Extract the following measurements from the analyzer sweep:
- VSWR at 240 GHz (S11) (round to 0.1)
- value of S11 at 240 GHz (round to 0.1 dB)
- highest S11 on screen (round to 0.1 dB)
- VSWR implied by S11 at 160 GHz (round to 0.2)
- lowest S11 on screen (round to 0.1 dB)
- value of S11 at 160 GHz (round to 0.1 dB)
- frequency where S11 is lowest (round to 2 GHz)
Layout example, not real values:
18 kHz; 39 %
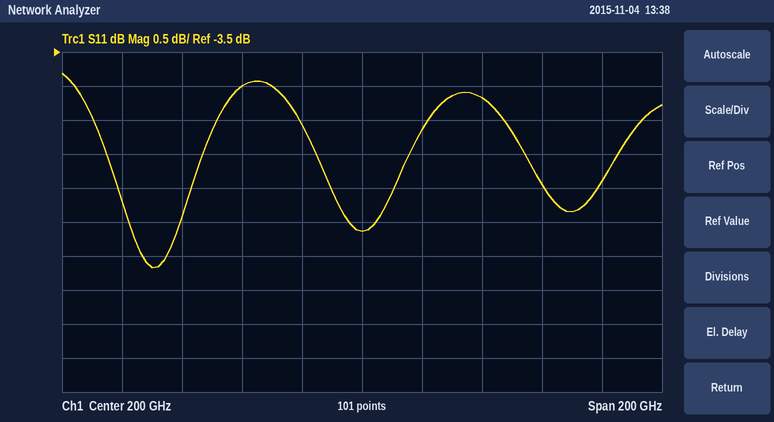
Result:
4.2; -4.2 dB; -3.8 dB; 4.4; -6.7 dB; -4.0 dB; 130 GHz
